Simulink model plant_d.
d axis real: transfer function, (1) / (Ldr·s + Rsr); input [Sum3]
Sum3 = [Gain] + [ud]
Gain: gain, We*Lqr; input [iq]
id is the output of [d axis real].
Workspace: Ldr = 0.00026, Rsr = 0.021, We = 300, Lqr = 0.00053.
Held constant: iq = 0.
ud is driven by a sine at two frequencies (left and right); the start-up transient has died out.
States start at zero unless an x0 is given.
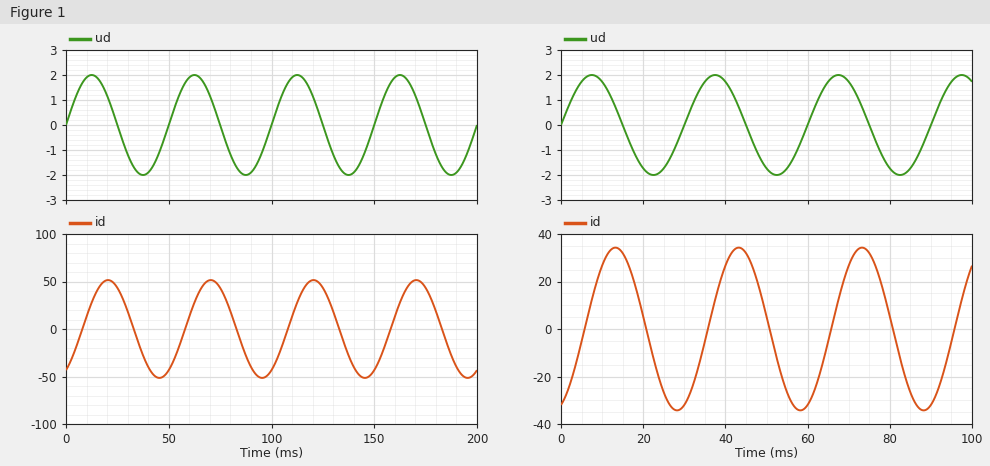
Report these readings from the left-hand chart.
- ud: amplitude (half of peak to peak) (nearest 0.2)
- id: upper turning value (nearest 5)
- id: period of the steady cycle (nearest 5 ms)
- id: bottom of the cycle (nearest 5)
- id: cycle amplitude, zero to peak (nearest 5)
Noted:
2.0
50
50 ms
-50
50
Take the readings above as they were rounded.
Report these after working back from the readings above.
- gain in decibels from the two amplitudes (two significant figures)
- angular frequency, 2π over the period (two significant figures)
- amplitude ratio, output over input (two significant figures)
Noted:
28 dB
0.13 rad/ms
25
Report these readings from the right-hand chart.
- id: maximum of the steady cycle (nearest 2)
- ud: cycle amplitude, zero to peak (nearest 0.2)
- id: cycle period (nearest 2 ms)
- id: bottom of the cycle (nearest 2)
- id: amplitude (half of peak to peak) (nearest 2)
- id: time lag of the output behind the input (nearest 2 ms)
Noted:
34
2.0
30 ms
-34
34
6 ms
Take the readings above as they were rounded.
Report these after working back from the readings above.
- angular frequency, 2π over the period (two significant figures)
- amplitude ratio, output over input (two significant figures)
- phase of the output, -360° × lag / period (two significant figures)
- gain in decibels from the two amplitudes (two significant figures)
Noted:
0.21 rad/ms
17
-72°
25 dB
